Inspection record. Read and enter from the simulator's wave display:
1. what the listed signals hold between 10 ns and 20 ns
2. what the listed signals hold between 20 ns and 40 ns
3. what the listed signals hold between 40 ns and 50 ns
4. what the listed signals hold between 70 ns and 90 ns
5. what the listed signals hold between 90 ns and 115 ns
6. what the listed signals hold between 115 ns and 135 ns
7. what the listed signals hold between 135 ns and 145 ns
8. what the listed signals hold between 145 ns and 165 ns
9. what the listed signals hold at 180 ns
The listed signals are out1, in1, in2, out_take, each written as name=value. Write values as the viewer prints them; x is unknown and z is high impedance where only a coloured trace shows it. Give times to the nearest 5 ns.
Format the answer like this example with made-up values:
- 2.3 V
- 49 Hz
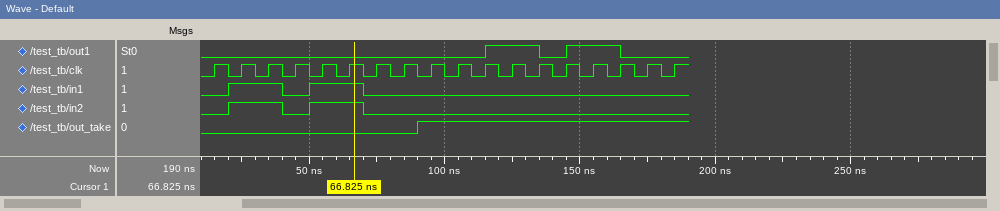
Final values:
- out1=0, in1=0, in2=0, out_take=0
- out1=0, in1=1, in2=1, out_take=0
- out1=0, in1=0, in2=0, out_take=0
- out1=0, in1=0, in2=0, out_take=0
- out1=0, in1=0, in2=0, out_take=1
- out1=1, in1=0, in2=0, out_take=1
- out1=0, in1=0, in2=0, out_take=1
- out1=1, in1=0, in2=0, out_take=1
- out1=0, in1=0, in2=0, out_take=1
